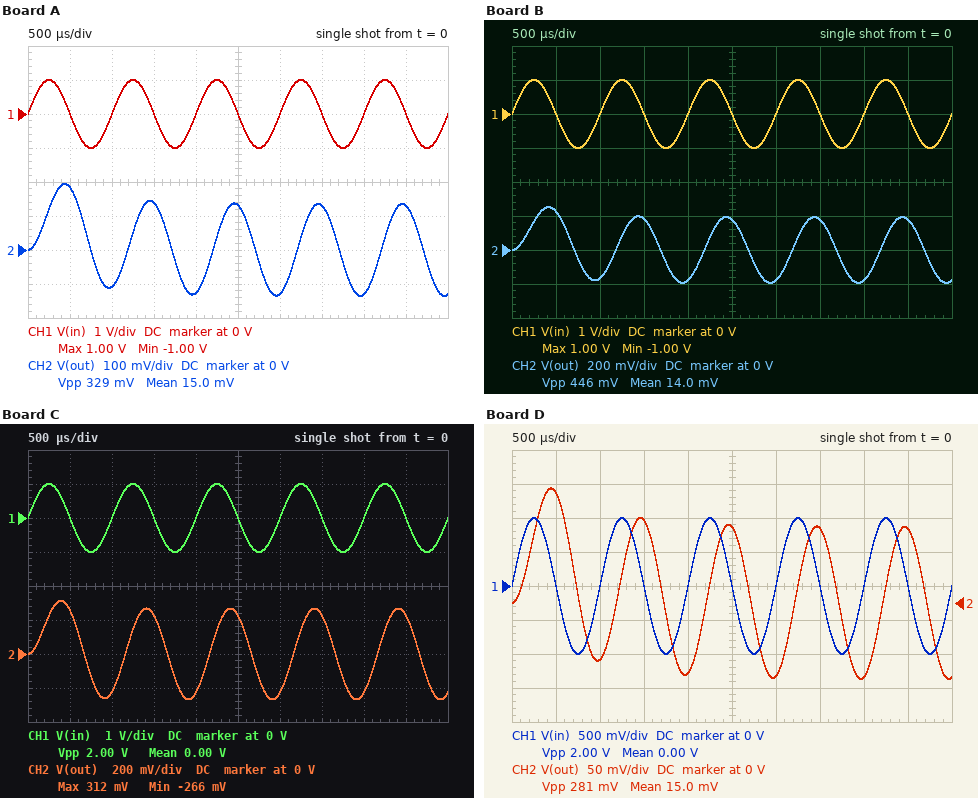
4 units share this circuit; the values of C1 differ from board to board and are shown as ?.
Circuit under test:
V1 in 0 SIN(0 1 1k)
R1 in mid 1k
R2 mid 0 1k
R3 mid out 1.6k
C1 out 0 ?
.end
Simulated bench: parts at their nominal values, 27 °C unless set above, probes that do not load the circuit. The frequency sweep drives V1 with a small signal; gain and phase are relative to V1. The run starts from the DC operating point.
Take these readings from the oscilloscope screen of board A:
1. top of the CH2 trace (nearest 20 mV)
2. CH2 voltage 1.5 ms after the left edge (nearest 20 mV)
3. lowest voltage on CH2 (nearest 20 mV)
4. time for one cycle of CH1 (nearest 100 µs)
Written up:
200 mV
140 mV
-140 mV
1.0 ms
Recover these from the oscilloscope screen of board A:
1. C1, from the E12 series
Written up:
270 nF
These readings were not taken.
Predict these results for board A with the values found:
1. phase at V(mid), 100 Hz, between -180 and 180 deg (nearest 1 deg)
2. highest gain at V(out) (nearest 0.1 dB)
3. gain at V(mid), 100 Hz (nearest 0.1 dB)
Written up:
-4 deg
-6.0 dB
-6.2 dB
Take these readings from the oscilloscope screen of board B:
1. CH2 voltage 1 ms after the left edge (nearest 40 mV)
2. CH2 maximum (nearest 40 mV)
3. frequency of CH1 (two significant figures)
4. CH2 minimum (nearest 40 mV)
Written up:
-160 mV
240 mV
1.0 kHz
-200 mV
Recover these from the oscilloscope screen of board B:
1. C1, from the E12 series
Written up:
180 nF
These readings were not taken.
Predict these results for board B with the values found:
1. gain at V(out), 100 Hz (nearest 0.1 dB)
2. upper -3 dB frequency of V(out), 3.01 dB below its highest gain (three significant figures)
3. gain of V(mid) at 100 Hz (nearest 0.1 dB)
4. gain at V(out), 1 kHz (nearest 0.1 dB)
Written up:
-6.3 dB
421 Hz
-6.1 dB
-14.2 dB
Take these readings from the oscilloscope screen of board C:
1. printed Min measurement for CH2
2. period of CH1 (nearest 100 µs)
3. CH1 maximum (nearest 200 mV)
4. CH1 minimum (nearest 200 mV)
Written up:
-266 mV
1.0 ms
1.0 V
-1.0 V
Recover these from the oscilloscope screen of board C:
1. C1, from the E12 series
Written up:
120 nF
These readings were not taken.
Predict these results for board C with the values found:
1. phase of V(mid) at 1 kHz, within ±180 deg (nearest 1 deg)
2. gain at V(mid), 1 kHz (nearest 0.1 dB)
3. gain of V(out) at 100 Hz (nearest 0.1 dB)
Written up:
-7 deg
-7.6 dB
-6.1 dB
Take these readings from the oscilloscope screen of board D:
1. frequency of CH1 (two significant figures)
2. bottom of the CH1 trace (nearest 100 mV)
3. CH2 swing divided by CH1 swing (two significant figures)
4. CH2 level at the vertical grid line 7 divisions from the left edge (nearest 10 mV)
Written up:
1.0 kHz
-1.0 V
0.14
110 mV
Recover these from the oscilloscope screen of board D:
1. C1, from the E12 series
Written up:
330 nF
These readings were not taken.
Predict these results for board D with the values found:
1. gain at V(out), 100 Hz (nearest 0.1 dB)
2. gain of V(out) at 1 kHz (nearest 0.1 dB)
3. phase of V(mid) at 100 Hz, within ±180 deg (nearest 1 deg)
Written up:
-6.8 dB
-19.0 dB
-5 deg
